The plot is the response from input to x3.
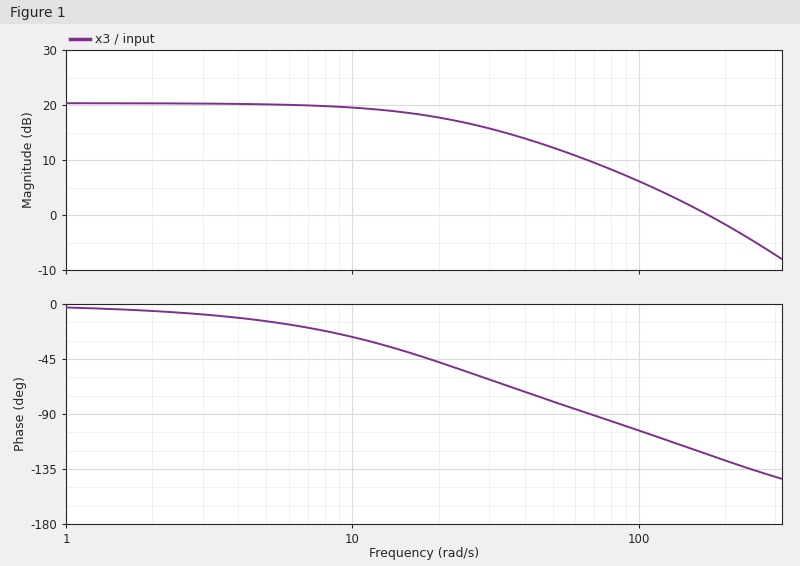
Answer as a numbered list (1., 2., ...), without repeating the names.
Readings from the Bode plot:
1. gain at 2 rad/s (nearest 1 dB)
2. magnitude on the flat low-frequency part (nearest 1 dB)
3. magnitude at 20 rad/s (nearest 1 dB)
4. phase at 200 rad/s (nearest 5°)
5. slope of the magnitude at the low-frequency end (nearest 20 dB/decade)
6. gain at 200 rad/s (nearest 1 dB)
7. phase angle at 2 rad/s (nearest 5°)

1. 20 dB
2. 20 dB
3. 18 dB
4. -130°
5. 0 dB/decade
6. -2 dB
7. -5°
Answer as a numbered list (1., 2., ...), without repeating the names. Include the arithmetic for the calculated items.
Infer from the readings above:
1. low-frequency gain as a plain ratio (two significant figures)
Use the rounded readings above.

1. 10^(20 / 20) = 10
